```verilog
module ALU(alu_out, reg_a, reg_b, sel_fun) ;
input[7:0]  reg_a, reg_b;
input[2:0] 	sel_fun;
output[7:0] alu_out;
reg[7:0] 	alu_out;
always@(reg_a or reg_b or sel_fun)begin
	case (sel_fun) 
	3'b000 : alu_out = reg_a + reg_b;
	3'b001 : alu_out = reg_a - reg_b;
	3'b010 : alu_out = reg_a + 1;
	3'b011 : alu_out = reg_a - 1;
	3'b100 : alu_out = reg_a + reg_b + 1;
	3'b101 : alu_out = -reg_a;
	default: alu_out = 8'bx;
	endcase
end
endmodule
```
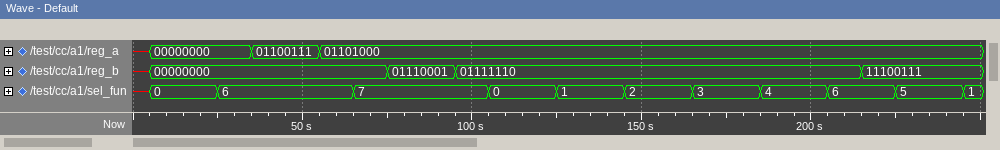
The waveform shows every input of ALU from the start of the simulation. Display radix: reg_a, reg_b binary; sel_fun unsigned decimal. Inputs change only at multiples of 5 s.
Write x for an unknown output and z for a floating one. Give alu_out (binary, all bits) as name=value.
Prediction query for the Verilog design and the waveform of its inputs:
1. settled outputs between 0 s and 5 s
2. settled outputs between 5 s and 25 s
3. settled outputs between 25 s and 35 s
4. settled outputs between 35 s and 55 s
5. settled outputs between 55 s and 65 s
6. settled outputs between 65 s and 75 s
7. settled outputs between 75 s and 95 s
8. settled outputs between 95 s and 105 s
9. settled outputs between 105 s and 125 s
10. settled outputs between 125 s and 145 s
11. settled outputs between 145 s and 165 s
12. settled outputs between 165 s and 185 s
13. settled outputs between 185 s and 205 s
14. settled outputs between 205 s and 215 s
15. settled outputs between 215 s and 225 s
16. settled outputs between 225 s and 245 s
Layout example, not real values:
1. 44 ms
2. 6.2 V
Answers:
1. alu_out=x
2. alu_out=00000000
3. alu_out=x
4. alu_out=x
5. alu_out=x
6. alu_out=x
7. alu_out=x
8. alu_out=x
9. alu_out=11100110
10. alu_out=11101010
11. alu_out=01101001
12. alu_out=01100111
13. alu_out=11100111
14. alu_out=x
15. alu_out=x
16. alu_out=10011000
